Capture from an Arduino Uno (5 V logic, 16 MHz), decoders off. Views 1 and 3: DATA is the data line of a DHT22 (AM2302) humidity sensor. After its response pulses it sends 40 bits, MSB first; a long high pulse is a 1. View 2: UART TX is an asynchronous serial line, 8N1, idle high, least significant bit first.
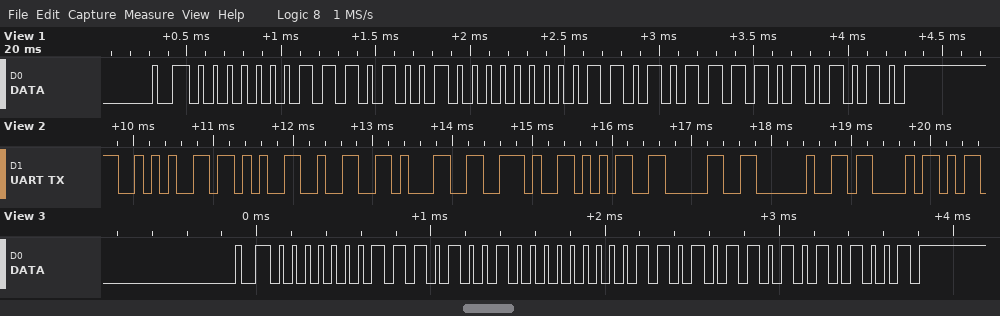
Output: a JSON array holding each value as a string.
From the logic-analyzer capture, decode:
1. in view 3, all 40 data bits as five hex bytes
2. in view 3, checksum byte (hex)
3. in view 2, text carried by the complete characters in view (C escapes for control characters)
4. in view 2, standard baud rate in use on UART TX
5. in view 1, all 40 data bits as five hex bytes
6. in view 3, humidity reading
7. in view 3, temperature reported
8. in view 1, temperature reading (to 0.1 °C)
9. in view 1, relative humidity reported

["01 D2 00 D6 A9", "0xA9", "\"*+21.50 C\"", "9600 baud", "01 D2 00 D7 AA", "46.6 %", "21.4 °C", "21.5 °C", "46.6 %"]
